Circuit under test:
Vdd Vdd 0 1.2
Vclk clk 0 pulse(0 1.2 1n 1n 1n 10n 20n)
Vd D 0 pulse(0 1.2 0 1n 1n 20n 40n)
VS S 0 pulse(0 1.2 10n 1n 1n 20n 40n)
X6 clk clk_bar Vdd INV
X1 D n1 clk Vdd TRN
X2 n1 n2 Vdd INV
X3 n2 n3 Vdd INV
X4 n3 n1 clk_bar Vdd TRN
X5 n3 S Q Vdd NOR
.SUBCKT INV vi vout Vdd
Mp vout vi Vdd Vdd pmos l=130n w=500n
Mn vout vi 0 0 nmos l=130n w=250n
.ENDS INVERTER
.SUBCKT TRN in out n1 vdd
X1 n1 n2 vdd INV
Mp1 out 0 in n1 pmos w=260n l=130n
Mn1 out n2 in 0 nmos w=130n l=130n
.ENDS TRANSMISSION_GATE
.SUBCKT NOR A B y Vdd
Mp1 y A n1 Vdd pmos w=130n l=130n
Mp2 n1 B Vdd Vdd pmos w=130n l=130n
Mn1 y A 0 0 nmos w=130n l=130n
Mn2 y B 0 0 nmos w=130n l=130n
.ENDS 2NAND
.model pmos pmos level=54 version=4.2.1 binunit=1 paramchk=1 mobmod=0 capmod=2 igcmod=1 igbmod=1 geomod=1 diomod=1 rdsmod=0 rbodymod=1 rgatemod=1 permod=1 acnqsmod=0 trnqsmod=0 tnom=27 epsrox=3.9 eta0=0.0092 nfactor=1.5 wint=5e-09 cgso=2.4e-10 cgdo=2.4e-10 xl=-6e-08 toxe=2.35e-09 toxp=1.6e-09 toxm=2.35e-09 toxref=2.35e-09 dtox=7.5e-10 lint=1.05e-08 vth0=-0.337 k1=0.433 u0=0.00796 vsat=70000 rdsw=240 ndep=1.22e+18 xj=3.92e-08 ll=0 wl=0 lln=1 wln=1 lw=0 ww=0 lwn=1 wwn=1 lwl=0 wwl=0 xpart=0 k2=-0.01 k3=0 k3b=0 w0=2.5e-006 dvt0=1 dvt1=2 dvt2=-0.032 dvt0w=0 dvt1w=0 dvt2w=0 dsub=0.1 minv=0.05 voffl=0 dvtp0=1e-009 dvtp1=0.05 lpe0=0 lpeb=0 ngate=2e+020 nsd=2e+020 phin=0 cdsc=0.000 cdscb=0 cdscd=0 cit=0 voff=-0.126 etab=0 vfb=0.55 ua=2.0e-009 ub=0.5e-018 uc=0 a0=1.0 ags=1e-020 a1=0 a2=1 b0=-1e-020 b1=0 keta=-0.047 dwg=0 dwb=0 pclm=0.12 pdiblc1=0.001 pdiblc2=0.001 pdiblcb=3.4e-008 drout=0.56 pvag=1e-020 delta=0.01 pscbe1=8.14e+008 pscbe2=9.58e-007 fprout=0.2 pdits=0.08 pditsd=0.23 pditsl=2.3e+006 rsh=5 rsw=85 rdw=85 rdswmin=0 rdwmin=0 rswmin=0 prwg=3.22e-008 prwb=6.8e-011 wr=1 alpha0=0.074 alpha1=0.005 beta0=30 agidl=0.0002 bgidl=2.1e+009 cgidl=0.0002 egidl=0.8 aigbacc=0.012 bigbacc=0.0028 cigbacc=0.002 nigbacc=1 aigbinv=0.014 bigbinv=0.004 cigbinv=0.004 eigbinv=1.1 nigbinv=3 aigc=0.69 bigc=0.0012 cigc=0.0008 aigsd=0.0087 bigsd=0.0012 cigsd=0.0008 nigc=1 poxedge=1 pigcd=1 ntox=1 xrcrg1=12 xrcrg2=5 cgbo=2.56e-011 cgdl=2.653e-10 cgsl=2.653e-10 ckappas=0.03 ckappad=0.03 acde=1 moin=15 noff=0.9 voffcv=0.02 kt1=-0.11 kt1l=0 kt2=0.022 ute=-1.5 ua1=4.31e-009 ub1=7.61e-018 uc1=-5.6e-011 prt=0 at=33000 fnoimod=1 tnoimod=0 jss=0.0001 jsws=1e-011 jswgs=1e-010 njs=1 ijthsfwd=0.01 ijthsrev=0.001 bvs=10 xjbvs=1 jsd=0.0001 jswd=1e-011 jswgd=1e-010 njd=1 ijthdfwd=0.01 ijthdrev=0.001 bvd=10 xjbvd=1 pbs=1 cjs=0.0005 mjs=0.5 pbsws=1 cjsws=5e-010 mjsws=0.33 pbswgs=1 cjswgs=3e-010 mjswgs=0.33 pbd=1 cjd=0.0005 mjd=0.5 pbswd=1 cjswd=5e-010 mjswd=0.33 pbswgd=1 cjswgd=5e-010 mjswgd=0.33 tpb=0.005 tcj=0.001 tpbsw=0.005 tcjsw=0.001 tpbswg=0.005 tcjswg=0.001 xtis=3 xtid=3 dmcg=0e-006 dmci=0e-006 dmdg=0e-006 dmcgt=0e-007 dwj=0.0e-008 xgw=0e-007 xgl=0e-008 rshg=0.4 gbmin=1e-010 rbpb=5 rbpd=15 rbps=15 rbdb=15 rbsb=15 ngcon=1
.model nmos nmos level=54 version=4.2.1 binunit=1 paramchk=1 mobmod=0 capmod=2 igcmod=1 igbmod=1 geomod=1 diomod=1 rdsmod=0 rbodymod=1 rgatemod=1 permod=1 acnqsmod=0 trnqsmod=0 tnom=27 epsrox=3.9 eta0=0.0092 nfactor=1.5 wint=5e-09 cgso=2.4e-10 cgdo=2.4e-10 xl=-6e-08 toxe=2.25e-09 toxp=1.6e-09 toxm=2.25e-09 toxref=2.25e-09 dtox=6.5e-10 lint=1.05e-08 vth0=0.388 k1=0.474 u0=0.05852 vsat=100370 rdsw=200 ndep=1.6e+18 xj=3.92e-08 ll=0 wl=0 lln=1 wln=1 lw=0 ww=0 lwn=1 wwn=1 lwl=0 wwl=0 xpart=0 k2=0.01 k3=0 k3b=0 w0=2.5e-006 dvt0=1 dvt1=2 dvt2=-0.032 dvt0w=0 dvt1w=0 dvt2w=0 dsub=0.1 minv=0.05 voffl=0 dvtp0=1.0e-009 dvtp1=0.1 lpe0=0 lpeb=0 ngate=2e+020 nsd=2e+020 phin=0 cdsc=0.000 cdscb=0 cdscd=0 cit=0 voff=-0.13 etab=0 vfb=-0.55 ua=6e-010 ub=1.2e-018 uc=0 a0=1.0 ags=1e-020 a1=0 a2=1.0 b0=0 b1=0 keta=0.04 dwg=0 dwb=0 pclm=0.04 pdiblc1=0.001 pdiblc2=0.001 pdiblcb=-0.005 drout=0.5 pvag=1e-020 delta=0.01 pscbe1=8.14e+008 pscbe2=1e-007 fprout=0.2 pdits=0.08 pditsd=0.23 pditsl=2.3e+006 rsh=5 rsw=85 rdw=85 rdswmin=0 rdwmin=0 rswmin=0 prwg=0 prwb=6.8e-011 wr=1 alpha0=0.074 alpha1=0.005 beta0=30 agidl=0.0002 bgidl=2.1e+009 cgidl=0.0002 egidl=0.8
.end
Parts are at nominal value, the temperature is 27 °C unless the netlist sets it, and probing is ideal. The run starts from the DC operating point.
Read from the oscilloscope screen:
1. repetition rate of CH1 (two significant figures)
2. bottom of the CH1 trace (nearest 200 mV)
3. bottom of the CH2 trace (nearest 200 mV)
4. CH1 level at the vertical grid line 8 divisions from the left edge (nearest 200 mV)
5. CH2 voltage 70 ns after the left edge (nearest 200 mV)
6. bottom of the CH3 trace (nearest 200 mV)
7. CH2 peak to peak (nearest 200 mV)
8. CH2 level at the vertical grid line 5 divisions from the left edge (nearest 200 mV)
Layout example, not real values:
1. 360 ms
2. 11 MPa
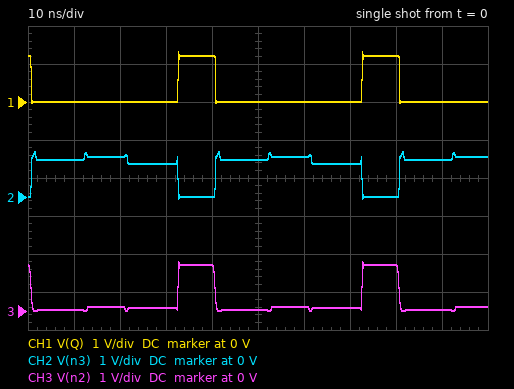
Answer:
1. 25 MHz
2. 0 V
3. 0 V
4. 1.2 V
5. 800 mV
6. 0 V
7. 1.2 V
8. 1.0 V
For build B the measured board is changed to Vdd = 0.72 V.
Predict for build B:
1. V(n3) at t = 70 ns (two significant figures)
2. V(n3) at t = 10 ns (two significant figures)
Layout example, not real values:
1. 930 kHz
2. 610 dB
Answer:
1. 650 mV
2. 710 mV
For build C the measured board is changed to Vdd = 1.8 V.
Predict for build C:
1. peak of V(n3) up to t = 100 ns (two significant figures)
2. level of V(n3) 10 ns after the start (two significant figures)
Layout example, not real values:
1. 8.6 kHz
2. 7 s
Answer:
1. 1.7 V
2. 1.4 V
